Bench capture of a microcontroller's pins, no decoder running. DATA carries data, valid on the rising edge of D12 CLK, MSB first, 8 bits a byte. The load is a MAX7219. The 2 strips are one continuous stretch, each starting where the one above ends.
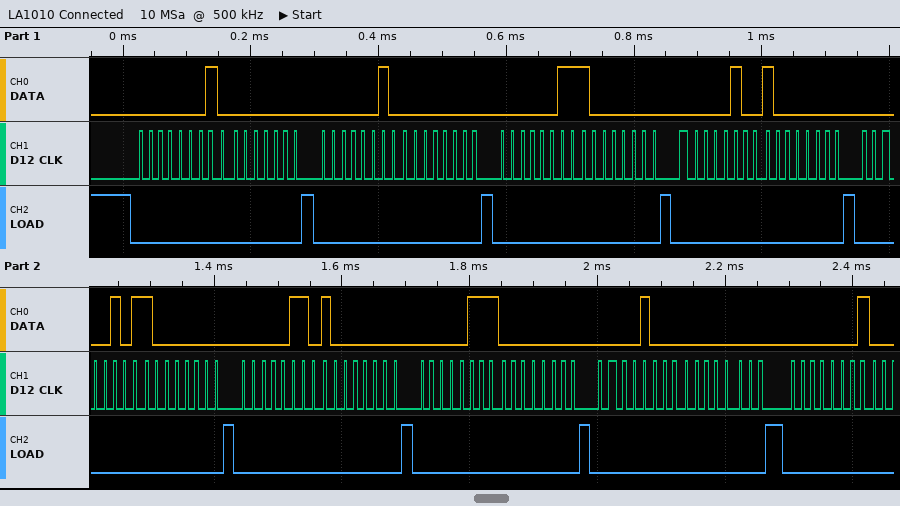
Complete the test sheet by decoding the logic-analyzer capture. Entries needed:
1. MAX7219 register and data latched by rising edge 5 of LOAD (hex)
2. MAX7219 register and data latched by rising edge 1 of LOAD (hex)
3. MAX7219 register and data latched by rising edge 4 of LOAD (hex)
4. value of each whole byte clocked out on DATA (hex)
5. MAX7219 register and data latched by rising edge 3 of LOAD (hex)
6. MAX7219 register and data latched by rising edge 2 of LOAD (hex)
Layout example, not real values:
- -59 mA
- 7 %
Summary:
- register 0x5, data 0x80
- register 0x1, data 0x00
- register 0x4, data 0x80
- 01 00 02 00 03 80 04 80 05 80 06 80 07 00 08 00 01
- register 0x3, data 0x80
- register 0x2, data 0x00
